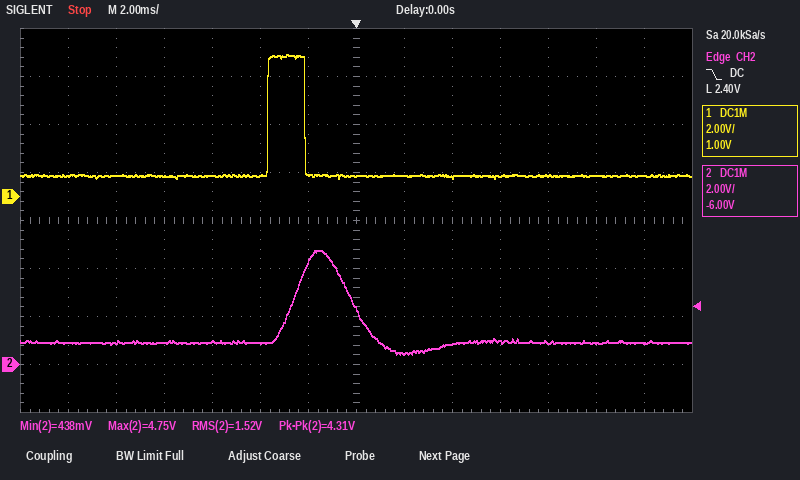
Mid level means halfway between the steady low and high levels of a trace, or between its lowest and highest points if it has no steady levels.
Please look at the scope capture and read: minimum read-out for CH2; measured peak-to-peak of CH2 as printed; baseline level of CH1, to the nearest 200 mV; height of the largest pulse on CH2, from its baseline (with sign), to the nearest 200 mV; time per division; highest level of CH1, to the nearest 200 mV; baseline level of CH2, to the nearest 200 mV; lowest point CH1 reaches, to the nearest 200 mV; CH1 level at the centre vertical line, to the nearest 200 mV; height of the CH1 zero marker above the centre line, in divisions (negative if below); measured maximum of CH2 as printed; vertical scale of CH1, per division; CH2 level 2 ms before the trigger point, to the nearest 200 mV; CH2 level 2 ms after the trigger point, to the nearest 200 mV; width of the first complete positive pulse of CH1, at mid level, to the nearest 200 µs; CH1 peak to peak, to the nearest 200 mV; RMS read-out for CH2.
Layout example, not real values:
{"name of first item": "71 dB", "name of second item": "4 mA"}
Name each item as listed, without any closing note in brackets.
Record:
{"minimum read-out for CH2": "438 mV", "measured peak-to-peak of CH2 as printed": "4.31 V", "baseline level of CH1, to the nearest 200 mV": "800 mV", "height of the largest pulse on CH2, from its baseline (with sign), to the nearest 200 mV": "+3.8 V", "time per division": "2 ms", "highest level of CH1, to the nearest 200 mV": "6.0 V", "baseline level of CH2, to the nearest 200 mV": "1.0 V", "lowest point CH1 reaches, to the nearest 200 mV": "800 mV", "CH1 level at the centre vertical line, to the nearest 200 mV": "800 mV", "height of the CH1 zero marker above the centre line, in divisions": "+0.5 div", "measured maximum of CH2 as printed": "4.75 V", "vertical scale of CH1, per division": "2 V", "CH2 level 2 ms before the trigger point, to the nearest 200 mV": "4.2 V", "CH2 level 2 ms after the trigger point, to the nearest 200 mV": "400 mV", "width of the first complete positive pulse of CH1, at mid level, to the nearest 200 µs": "1.6 ms", "CH1 peak to peak, to the nearest 200 mV": "5.2 V", "RMS read-out for CH2": "1.52 V"}
